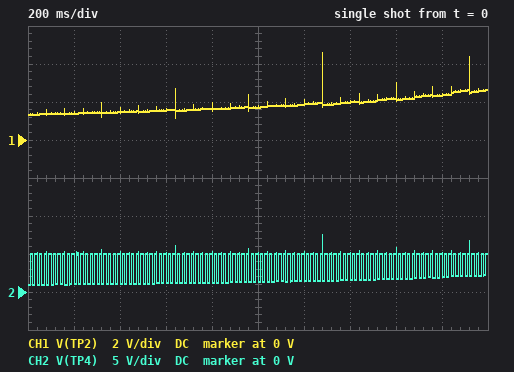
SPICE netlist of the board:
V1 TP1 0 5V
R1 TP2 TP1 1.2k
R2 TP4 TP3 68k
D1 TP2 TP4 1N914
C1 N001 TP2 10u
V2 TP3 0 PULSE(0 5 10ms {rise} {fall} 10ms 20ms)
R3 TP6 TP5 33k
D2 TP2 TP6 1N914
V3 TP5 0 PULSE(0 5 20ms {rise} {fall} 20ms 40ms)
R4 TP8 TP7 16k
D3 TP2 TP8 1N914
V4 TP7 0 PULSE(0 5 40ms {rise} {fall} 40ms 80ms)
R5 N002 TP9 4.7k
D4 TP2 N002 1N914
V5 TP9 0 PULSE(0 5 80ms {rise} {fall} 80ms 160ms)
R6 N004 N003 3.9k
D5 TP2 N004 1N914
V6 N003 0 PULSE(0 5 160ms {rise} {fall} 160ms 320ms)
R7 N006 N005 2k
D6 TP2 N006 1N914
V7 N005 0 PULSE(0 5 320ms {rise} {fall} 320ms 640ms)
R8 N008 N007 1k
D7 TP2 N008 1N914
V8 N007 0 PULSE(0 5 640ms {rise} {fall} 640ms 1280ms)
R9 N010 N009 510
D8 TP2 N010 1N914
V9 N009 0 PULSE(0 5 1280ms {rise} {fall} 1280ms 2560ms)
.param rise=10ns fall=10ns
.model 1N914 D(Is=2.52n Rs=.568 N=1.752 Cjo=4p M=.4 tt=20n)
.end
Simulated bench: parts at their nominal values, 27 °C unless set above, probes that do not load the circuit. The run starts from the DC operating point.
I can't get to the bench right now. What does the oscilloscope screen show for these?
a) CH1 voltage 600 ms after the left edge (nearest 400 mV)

1.6 V
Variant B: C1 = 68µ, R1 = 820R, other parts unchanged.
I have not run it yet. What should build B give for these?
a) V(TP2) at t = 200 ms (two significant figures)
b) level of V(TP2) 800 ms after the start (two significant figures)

1.7 V
2.0 V
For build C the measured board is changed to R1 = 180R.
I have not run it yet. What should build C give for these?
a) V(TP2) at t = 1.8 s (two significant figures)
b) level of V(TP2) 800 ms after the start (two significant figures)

4.2 V
3.6 V
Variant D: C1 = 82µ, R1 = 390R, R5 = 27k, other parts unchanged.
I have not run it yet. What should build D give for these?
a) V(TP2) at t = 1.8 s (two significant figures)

3.7 V
